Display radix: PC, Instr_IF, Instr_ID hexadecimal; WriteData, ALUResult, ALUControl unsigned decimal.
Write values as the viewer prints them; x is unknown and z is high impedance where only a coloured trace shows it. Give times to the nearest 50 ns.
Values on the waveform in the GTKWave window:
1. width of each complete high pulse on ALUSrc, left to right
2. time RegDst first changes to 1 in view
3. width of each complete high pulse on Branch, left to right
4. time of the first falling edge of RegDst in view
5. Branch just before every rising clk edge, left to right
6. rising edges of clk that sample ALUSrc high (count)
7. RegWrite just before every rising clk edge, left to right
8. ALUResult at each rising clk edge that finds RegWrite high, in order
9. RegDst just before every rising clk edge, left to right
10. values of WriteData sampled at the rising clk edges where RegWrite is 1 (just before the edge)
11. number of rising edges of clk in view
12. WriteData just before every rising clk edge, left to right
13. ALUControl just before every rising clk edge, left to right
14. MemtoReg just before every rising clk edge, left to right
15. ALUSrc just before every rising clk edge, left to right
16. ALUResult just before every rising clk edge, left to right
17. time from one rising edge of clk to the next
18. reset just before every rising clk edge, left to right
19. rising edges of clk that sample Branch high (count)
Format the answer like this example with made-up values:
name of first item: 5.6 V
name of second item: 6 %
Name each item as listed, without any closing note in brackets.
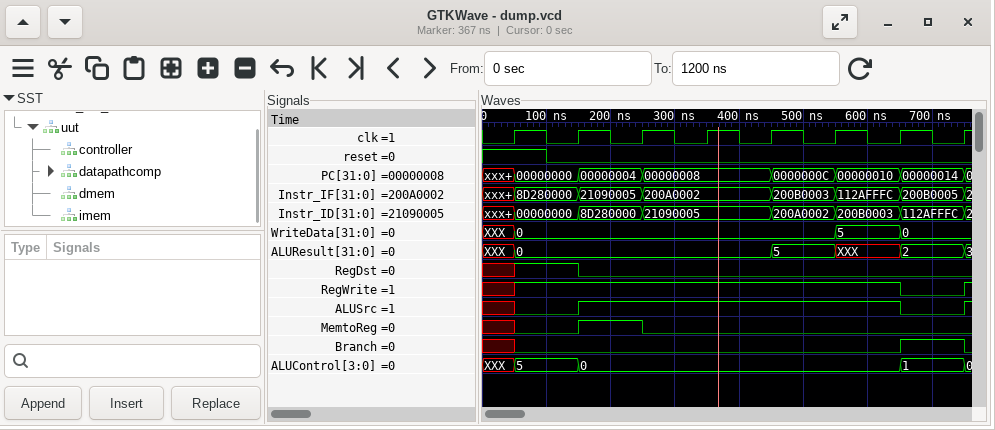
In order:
width of each complete high pulse on ALUSrc, left to right: 500 ns
time RegDst first changes to 1 in view: 50 ns
width of each complete high pulse on Branch, left to right: 100 ns
time of the first falling edge of RegDst in view: 150 ns
Branch just before every rising clk edge, left to right: x 0 0 0 0 0 0 1
rising edges of clk that sample ALUSrc high: 5
RegWrite just before every rising clk edge, left to right: x 1 1 1 1 1 1 0
ALUResult at each rising clk edge that finds RegWrite high, in order: 0, 0, 0, 0, 5, XXX
RegDst just before every rising clk edge, left to right: x 1 0 0 0 0 0 0
values of WriteData sampled at the rising clk edges where RegWrite is 1: 0, 0, 0, 0, 0, 5
number of rising edges of clk in view: 8
WriteData just before every rising clk edge, left to right: XXX, 0, 0, 0, 0, 0, 5, 0
ALUControl just before every rising clk edge, left to right: XXX, 5, 0, 0, 0, 0, 0, 1
MemtoReg just before every rising clk edge, left to right: x 0 1 0 0 0 0 0
ALUSrc just before every rising clk edge, left to right: x 0 1 1 1 1 1 0
ALUResult just before every rising clk edge, left to right: XXX, 0, 0, 0, 0, 5, XXX, 2
time from one rising edge of clk to the next: 100 ns
reset just before every rising clk edge, left to right: 1 0 0 0 0 0 0 0
rising edges of clk that sample Branch high: 1
